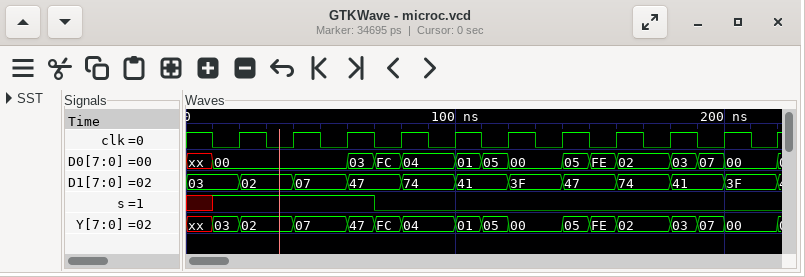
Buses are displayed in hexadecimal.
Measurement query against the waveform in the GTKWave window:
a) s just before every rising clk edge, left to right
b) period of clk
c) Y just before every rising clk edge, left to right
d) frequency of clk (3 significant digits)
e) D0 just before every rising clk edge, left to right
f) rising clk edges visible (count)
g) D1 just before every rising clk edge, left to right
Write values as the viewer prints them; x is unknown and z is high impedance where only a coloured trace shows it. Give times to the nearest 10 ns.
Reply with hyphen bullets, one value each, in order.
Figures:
- 1 1 1 0 0 0 0 0 0 0 0
- 20 ns
- 03, 02, 07, FC, 04, 05, 00, FE, 02, 07, 00
- 50.0 MHz
- 00, 00, 00, FC, 04, 05, 00, FE, 02, 07, 00
- 11
- 03, 02, 07, 47, 74, 41, 3F, 47, 74, 41, 3F
